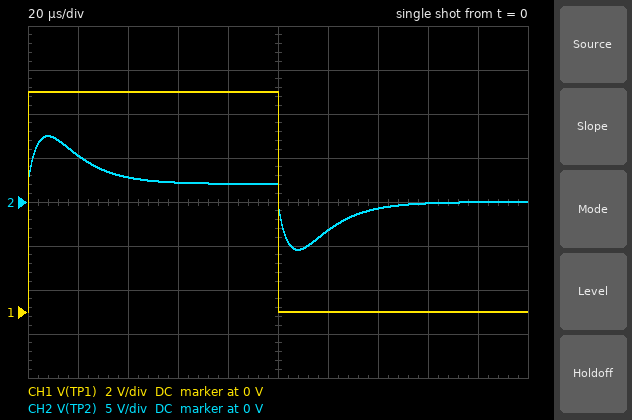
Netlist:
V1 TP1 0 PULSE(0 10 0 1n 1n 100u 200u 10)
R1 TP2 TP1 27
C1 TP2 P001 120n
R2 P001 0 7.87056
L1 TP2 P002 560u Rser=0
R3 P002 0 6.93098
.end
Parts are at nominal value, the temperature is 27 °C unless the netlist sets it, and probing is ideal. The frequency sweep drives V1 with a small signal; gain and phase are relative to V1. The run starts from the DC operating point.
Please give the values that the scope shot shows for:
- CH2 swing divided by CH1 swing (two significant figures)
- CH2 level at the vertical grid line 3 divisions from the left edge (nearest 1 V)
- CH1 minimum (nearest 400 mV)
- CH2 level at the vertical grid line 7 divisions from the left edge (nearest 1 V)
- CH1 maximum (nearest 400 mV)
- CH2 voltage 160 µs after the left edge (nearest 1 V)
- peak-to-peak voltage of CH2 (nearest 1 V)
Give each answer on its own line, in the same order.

1.3
2 V
0 V
-1 V
10.0 V
0 V
13 V
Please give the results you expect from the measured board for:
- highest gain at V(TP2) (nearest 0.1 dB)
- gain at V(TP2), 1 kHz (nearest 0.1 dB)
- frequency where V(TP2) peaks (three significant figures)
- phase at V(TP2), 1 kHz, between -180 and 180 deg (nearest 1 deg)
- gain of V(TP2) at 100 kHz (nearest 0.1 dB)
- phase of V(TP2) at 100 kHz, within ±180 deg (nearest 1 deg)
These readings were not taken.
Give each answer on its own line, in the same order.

-0.7 dB
-12.8 dB
19.2 kHz
21 deg
-7.5 dB
-37 deg
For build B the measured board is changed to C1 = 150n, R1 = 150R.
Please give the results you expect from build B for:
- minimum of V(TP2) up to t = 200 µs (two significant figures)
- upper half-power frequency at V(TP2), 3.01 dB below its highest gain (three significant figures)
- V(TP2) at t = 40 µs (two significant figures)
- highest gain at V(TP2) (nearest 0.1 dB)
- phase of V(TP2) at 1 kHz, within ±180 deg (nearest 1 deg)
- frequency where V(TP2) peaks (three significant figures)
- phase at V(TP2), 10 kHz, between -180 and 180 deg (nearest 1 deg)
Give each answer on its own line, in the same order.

-2.5 V
23.6 kHz
-390 mV
-4.0 dB
25 deg
17.3 kHz
55 deg
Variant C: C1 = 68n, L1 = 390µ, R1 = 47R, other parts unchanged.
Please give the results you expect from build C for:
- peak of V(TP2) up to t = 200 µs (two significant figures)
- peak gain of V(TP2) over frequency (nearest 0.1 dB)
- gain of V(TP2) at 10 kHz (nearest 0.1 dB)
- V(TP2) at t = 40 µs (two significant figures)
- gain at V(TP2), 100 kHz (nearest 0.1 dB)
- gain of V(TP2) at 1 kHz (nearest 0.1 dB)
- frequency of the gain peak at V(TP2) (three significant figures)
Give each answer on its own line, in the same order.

6.4 V
-1.0 dB
-6.8 dB
1.2 V
-7.2 dB
-17.3 dB
30.7 kHz
